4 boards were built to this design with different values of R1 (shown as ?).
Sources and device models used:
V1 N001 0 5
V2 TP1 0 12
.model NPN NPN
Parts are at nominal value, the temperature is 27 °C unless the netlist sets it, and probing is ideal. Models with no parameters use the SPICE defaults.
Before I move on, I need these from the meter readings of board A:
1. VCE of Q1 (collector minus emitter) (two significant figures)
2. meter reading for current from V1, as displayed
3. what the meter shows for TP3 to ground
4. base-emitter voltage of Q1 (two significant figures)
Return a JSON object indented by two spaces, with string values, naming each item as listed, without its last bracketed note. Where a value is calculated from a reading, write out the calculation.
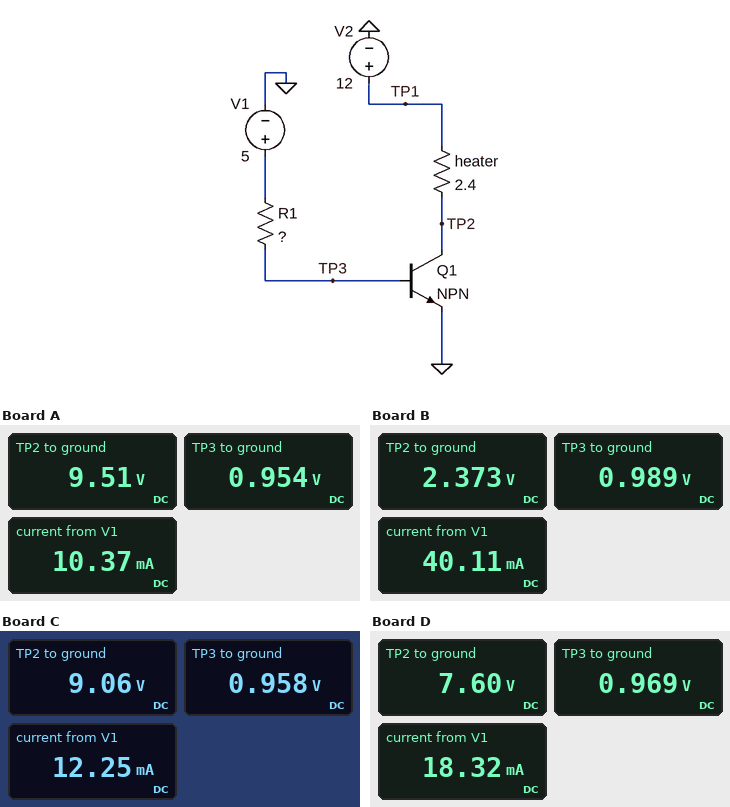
{
  "VCE of Q1 (collector minus emitter)": "9.51 V = 9.5 V",
  "meter reading for current from V1, as displayed": "10.37 mA",
  "what the meter shows for TP3 to ground": "0.954 V",
  "base-emitter voltage of Q1": "954 mV = 950 mV"
}
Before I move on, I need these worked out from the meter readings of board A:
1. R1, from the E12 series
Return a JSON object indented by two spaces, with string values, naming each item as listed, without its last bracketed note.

{
  "R1, from the E12 series": "390 Ω"
}
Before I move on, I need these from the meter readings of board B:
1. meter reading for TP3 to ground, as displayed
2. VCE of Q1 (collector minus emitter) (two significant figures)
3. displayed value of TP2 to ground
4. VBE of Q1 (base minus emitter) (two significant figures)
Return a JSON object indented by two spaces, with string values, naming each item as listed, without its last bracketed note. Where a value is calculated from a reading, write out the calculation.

{
  "meter reading for TP3 to ground, as displayed": "0.989 V",
  "VCE of Q1 (collector minus emitter)": "2.373 V = 2.4 V",
  "displayed value of TP2 to ground": "2.373 V",
  "VBE of Q1 (base minus emitter)": "989 mV = 990 mV"
}
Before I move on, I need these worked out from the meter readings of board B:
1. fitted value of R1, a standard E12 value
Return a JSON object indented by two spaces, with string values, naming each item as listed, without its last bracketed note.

{
  "fitted value of R1, a standard E12 value": "100 Ω"
}
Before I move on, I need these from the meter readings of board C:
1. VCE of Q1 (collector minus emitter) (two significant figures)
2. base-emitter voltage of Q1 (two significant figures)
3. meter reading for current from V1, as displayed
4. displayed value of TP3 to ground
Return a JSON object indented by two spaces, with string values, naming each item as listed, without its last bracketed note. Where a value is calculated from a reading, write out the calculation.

{
  "VCE of Q1 (collector minus emitter)": "9.06 V = 9.1 V",
  "base-emitter voltage of Q1": "958 mV = 960 mV",
  "meter reading for current from V1, as displayed": "12.25 mA",
  "displayed value of TP3 to ground": "0.958 V"
}
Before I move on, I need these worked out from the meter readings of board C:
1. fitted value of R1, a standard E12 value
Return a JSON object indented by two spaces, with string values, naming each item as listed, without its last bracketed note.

{
  "fitted value of R1, a standard E12 value": "330 Ω"
}
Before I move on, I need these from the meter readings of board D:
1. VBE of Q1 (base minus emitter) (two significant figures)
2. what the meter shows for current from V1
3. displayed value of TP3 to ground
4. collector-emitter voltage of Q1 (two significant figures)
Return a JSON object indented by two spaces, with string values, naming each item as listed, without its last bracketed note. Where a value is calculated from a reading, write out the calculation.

{
  "VBE of Q1 (base minus emitter)": "969 mV = 970 mV",
  "what the meter shows for current from V1": "18.32 mA",
  "displayed value of TP3 to ground": "0.969 V",
  "collector-emitter voltage of Q1": "7.6 V = 7.6 V"
}
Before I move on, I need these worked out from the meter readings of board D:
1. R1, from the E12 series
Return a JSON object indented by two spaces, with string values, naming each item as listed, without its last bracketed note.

{
  "R1, from the E12 series": "220 Ω"
}
